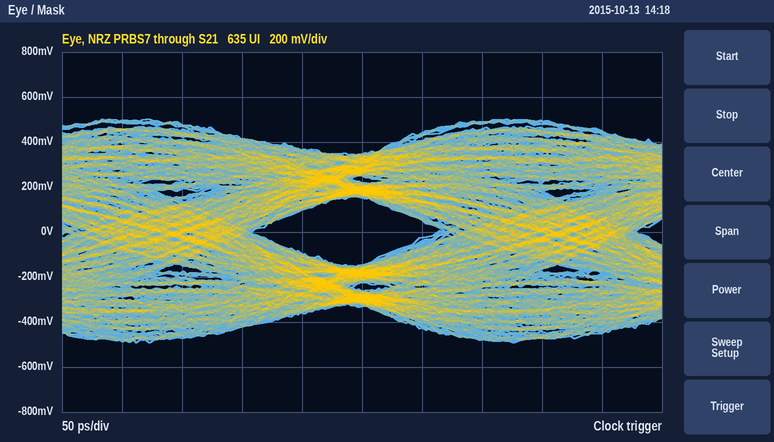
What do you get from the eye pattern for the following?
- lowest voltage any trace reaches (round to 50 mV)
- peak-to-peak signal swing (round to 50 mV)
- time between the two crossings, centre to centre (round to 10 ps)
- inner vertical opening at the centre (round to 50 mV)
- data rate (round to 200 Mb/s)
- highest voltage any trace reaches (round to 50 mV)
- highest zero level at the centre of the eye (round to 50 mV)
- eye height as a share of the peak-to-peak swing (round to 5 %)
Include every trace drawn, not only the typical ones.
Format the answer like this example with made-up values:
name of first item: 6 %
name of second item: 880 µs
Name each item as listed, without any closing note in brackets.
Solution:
lowest voltage any trace reaches: -500 mV
peak-to-peak signal swing: 1.00 V
time between the two crossings, centre to centre: 320 ps
inner vertical opening at the centre: 300 mV
data rate: 3.2 Gb/s
highest voltage any trace reaches: 500 mV
highest zero level at the centre of the eye: -150 mV
eye height as a share of the peak-to-peak swing: 30 %
